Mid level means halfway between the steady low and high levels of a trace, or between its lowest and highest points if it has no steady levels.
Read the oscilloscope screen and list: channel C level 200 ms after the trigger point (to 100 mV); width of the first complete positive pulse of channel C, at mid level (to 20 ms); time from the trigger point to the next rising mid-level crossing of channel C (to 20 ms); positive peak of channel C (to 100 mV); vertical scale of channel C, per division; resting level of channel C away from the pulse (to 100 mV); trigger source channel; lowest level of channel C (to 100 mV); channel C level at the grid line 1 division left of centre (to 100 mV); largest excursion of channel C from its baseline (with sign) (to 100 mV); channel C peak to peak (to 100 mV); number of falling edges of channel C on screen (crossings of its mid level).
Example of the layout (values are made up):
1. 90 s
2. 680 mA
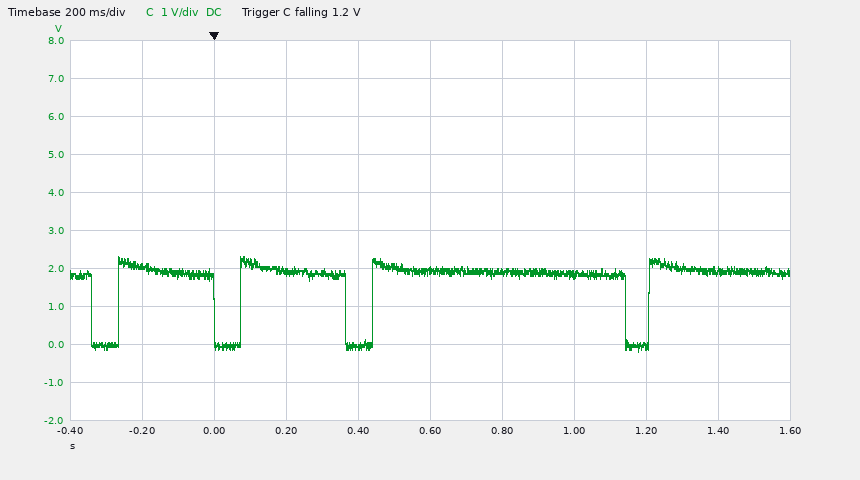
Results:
1. 1.9 V
2. 260 ms
3. 80 ms
4. 2.3 V
5. 1 V
6. 1.9 V
7. channel C
8. -200 mV
9. 0.0 V
10. -2.1 V
11. 2.5 V
12. 4
